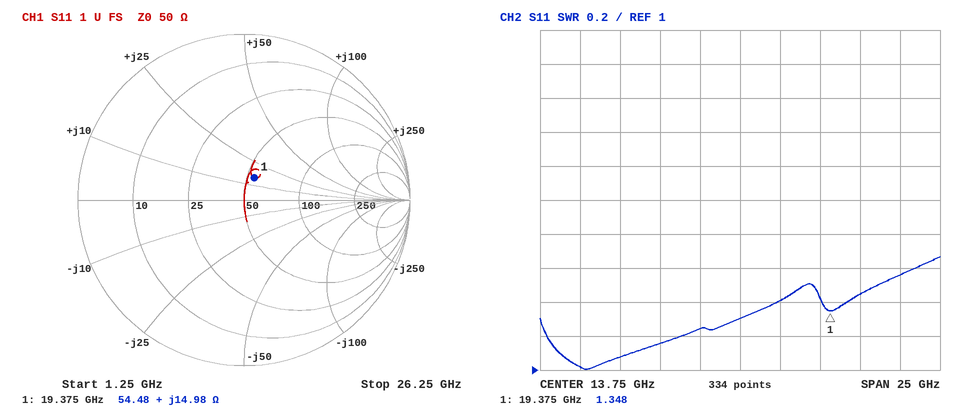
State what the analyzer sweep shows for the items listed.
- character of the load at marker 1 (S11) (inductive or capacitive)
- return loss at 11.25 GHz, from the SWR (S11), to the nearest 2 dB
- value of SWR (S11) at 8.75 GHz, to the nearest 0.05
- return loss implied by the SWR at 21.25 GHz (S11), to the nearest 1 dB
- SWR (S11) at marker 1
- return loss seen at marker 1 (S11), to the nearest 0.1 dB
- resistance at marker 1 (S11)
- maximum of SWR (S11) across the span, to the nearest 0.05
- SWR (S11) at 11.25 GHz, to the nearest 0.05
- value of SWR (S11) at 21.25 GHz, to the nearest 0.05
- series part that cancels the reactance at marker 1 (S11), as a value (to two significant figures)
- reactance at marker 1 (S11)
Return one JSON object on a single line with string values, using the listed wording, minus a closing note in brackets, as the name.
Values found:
{"character of the load at marker 1 (S11)": "inductive", "return loss at 11.25 GHz, from the SWR (S11), to the nearest 2 dB": "20 dB", "value of SWR (S11) at 8.75 GHz, to the nearest 0.05": "1.15", "return loss implied by the SWR at 21.25 GHz (S11), to the nearest 1 dB": "15 dB", "SWR (S11) at marker 1": "1.348", "return loss seen at marker 1 (S11), to the nearest 0.1 dB": "16.6 dB", "resistance at marker 1": "54.48 Ω", "maximum of SWR (S11) across the span, to the nearest 0.05": "1.65", "SWR (S11) at 11.25 GHz, to the nearest 0.05": "1.25", "value of SWR (S11) at 21.25 GHz, to the nearest 0.05": "1.45", "series part that cancels the reactance at marker 1 (S11), as a value": "550 fF", "reactance at marker 1": "+14.98 Ω"}
